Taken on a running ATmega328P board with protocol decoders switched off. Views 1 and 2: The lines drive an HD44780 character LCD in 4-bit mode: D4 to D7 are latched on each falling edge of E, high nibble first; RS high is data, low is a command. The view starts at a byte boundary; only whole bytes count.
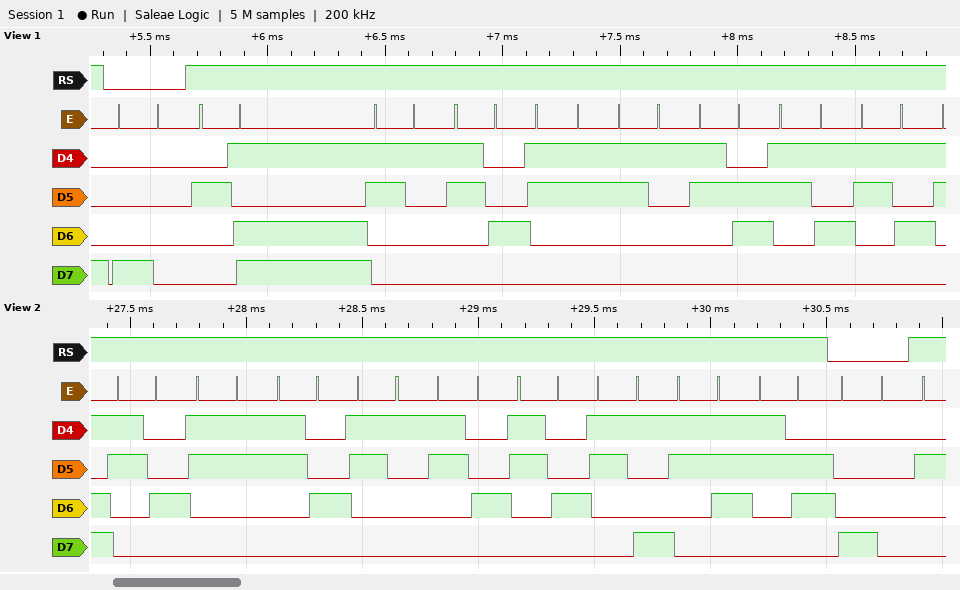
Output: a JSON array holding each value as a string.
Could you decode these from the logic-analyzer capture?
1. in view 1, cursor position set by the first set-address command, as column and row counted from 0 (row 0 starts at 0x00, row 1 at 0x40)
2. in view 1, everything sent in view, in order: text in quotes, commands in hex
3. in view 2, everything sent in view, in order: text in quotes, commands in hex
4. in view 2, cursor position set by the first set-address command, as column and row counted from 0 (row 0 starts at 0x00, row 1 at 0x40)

["column 0, row 0", "0x80 \"-1431655\"", "\"434144976\" 0x80", "column 0, row 0"]
